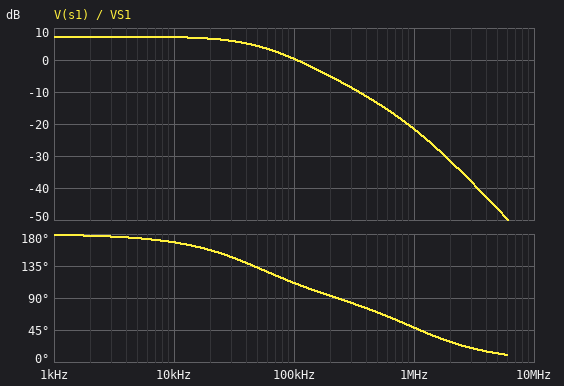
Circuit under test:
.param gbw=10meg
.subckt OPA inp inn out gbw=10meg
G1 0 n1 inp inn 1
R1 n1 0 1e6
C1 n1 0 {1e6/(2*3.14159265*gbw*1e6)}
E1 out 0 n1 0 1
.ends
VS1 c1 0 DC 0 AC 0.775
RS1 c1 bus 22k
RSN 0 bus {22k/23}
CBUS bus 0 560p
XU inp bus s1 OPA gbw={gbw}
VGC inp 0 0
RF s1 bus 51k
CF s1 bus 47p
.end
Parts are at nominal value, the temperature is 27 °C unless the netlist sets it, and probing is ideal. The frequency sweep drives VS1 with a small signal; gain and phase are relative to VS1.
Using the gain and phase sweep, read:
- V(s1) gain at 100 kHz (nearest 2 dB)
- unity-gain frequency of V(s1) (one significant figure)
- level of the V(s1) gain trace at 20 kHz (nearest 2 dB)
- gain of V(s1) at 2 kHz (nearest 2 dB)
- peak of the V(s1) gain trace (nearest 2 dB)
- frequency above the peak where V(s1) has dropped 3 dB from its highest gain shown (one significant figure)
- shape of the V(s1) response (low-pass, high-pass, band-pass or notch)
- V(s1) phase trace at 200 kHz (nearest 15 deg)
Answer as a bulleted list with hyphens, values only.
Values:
- 0 dB
- 100 kHz
- 6 dB
- 8 dB
- 8 dB
- 50 kHz
- low-pass
- 90 deg
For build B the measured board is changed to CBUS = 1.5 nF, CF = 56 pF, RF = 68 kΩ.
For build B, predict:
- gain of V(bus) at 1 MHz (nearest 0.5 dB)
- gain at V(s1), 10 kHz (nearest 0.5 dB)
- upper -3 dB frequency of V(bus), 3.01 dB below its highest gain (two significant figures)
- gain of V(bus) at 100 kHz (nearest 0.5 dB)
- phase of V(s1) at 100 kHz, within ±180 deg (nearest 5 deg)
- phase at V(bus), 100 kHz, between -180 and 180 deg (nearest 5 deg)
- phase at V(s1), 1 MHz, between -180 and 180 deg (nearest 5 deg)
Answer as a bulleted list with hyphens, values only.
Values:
- -47.5 dB
- 9.5 dB
- 500 kHz
- -40.0 dB
- 95 deg
- 5 deg
- 25 deg
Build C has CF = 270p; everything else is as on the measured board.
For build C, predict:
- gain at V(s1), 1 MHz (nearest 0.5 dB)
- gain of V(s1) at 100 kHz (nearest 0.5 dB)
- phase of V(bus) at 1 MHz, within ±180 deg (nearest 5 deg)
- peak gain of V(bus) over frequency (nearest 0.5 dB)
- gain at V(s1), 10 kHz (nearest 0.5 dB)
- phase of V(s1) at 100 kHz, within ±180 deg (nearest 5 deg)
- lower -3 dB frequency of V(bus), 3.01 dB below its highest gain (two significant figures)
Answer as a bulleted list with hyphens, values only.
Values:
- -32.5 dB
- -12.0 dB
- -15 deg
- -52.0 dB
- 4.5 dB
- 95 deg
- 11 kHz
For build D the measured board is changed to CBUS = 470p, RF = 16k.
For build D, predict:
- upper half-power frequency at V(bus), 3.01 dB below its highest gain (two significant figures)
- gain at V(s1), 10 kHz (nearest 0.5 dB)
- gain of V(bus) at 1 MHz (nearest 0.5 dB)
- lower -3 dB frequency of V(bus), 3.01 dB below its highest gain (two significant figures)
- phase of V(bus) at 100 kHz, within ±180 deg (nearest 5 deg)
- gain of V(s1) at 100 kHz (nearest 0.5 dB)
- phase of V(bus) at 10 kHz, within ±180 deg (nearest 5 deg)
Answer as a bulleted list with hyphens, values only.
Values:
- 1.4 MHz
- -3.0 dB
- -40.5 dB
- 140 kHz
- 55 deg
- -4.0 dB
- 85 deg
